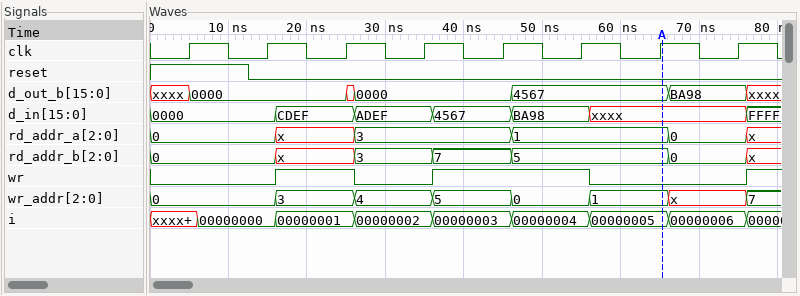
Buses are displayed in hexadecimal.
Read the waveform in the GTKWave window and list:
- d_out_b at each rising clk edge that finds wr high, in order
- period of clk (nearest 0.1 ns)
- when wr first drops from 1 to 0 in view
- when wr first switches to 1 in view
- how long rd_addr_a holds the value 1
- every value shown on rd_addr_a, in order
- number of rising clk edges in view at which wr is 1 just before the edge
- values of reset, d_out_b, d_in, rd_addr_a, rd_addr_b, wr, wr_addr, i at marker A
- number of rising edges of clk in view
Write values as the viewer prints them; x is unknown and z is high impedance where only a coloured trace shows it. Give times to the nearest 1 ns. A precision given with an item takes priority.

0000, 0000, 4567
10 ns
26 ns
16 ns
20 ns
0, x, 3, 1, 0, x
3
reset=0, d_out_b=4567, d_in=xxxx, rd_addr_a=1, rd_addr_b=5, wr=0, wr_addr=1, i=00000005
8
